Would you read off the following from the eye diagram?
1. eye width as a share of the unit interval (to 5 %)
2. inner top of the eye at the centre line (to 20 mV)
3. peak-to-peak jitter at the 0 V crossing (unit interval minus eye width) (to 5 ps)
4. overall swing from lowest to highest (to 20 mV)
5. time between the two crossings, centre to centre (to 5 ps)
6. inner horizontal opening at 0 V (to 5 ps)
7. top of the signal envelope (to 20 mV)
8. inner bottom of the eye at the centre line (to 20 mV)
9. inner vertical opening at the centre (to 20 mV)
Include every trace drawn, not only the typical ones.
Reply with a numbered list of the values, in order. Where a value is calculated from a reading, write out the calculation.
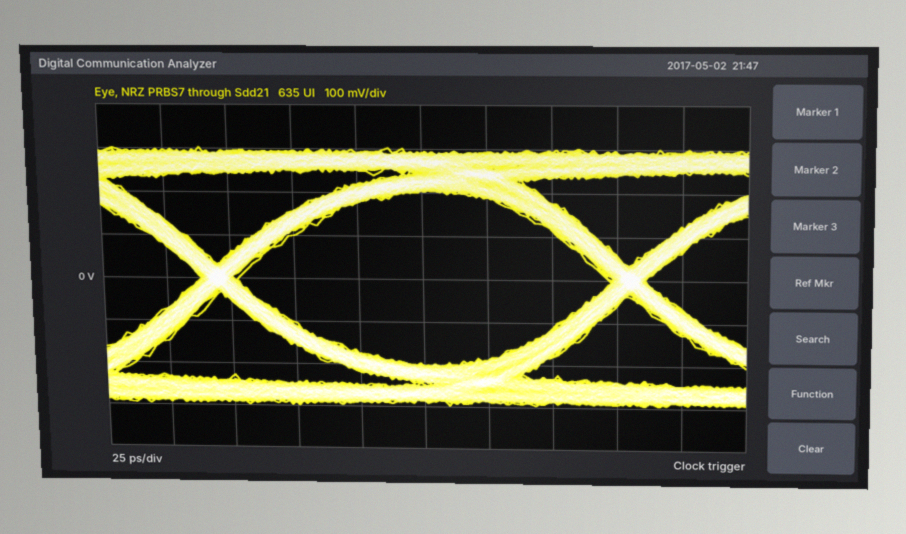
1. 145 ps / 160 ps ≈ 90.6 %, so 90 % to the nearest 5 %
2. 200 mV
3. 15 ps
4. 600 mV
5. 160 ps
6. 145 ps
7. 300 mV
8. -200 mV
9. 400 mV
